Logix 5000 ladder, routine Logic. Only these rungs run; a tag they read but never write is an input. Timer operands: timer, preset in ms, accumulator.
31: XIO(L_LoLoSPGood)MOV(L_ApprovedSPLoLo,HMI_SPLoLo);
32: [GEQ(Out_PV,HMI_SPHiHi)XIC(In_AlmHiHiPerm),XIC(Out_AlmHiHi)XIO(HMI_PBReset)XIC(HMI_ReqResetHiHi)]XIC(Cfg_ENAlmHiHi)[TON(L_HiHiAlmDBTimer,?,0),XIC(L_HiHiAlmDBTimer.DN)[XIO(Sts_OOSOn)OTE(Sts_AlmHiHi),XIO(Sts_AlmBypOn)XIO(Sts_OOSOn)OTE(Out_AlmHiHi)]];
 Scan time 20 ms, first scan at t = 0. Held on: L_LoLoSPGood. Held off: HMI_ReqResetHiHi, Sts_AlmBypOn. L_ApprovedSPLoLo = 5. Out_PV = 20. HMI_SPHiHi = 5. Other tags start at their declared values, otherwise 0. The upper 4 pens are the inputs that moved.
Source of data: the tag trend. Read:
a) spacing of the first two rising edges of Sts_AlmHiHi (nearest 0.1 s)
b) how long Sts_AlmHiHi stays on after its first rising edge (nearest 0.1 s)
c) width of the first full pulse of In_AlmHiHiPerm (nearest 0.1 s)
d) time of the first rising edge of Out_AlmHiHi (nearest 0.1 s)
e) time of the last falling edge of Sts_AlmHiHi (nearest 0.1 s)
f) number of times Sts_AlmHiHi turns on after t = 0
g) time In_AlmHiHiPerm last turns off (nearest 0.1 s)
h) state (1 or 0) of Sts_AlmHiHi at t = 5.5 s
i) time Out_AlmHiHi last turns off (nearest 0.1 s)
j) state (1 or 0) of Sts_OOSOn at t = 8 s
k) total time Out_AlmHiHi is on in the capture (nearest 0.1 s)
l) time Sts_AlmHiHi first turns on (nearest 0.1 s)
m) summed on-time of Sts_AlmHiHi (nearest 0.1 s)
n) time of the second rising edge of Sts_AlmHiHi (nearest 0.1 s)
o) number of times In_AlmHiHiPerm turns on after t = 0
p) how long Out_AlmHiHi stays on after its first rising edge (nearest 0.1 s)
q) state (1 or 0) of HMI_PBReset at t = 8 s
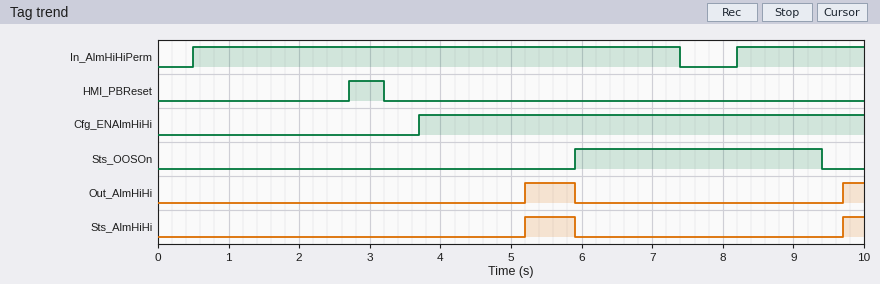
4.5 s
0.7 s
6.9 s
5.2 s
5.9 s
2
7.4 s
1
5.9 s
1
1.0 s
5.2 s
1.0 s
9.7 s
2
0.7 s
0
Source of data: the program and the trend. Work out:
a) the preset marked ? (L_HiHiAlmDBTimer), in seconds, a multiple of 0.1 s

1.5 s
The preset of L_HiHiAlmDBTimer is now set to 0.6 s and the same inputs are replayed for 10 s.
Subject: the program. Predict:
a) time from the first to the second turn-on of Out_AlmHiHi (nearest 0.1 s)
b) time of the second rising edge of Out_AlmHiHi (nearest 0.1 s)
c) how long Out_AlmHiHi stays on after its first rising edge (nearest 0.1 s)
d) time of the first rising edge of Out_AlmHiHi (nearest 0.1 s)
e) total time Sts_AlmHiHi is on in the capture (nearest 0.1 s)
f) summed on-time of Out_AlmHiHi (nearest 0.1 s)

5.1 s
9.4 s
1.6 s
4.3 s
2.2 s
2.2 s
